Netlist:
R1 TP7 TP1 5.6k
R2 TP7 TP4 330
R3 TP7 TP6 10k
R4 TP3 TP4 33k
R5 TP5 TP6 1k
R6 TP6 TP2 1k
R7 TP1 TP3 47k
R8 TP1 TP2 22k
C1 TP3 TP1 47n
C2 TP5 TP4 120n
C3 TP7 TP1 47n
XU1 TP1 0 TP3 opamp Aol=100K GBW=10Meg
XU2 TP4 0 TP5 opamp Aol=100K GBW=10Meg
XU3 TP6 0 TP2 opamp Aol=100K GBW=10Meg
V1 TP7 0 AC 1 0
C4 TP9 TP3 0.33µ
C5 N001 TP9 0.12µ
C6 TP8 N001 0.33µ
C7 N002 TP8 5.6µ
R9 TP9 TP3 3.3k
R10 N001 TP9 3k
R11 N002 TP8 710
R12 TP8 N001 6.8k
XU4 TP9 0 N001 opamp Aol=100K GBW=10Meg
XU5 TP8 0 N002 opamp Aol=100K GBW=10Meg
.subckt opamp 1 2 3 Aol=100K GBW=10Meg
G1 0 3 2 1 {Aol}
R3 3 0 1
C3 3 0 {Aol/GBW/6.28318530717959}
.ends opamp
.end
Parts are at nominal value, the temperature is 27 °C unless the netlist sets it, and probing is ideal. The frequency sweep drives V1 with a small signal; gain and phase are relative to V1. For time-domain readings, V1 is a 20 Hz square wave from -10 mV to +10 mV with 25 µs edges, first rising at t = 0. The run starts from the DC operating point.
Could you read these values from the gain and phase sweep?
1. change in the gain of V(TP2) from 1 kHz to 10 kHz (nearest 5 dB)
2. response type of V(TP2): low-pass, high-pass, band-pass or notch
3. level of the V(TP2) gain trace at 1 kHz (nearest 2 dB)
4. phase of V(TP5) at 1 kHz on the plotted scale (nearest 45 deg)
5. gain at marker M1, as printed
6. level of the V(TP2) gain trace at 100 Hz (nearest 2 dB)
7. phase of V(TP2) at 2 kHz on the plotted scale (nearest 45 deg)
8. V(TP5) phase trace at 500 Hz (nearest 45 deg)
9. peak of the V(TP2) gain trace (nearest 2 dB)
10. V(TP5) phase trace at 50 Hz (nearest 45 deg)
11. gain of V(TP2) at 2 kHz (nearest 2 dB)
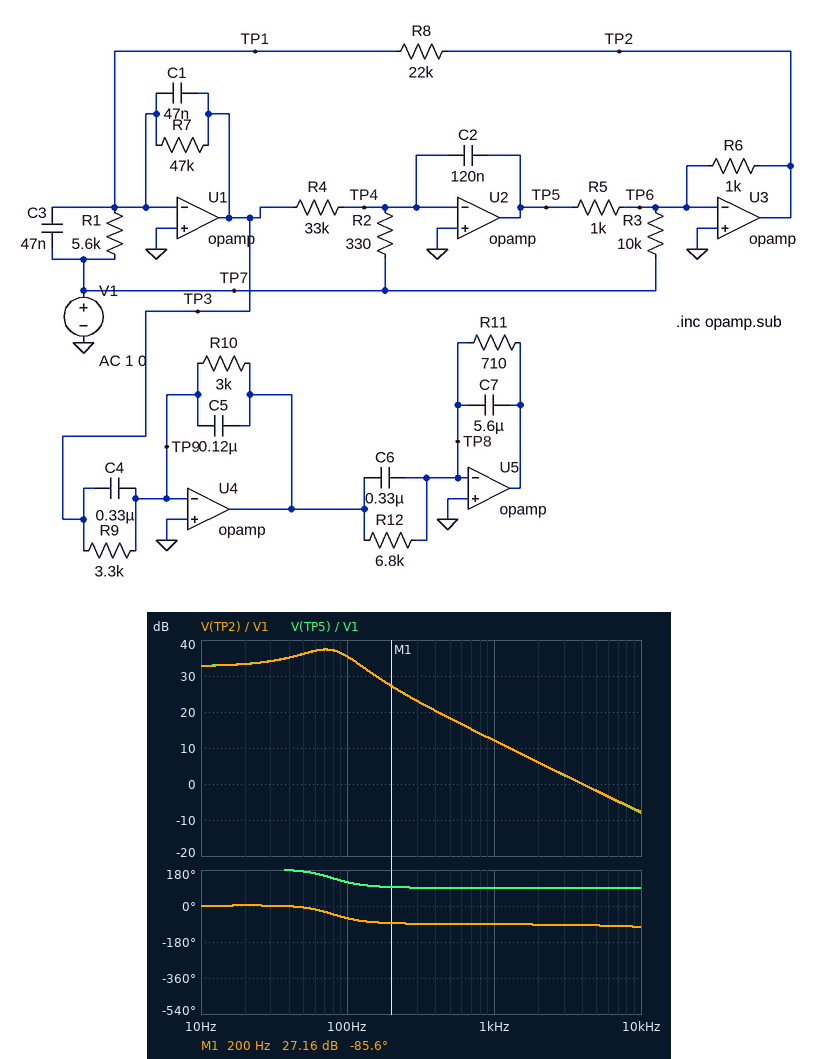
-20 dB
low-pass
12 dB
90 deg
27.16 dB
36 dB
-90 deg
90 deg
38 dB
180 deg
6 dB
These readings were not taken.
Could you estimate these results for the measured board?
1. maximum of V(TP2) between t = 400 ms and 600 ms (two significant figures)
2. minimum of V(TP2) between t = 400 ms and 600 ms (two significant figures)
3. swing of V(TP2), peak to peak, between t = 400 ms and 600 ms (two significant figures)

780 mV
-780 mV
1.6 V
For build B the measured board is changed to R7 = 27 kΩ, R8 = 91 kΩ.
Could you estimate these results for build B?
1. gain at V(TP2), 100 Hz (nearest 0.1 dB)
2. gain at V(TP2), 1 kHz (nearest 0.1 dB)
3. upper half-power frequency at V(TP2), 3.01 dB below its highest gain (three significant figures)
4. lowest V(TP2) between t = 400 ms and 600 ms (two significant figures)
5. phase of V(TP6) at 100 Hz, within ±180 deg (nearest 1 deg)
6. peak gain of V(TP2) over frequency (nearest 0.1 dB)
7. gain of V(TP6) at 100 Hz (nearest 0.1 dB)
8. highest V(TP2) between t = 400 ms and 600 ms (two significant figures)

32.3 dB
12.0 dB
13.4 Hz
-2.5 V
140 deg
50.1 dB
-64.7 dB
2.5 V
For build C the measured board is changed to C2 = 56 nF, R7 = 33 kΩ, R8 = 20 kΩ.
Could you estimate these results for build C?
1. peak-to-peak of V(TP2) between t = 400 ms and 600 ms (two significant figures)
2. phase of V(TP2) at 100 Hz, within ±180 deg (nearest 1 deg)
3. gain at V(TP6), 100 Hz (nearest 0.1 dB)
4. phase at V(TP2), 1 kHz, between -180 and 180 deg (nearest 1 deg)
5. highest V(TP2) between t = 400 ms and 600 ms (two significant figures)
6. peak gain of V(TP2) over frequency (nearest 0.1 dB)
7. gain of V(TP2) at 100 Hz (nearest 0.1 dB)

2.2 V
-20 deg
-56.5 dB
-90 deg
1.1 V
40.7 dB
40.5 dB
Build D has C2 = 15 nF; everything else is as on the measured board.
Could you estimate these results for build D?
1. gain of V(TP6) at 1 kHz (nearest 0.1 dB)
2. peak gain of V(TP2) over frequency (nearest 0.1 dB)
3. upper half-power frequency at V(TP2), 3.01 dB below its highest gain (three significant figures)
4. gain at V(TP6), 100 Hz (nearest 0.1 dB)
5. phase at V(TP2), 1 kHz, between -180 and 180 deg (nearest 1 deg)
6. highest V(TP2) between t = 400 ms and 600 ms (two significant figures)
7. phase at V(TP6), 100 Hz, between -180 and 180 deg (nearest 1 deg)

-49.5 dB
53.2 dB
260 Hz
-57.4 dB
-90 deg
2.6 V
-89 deg
